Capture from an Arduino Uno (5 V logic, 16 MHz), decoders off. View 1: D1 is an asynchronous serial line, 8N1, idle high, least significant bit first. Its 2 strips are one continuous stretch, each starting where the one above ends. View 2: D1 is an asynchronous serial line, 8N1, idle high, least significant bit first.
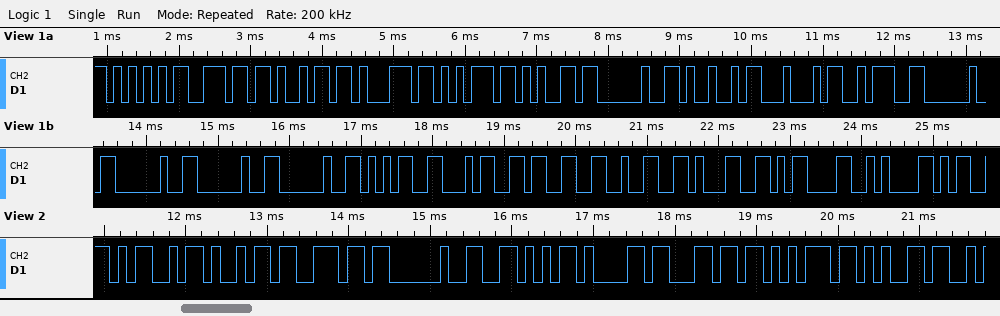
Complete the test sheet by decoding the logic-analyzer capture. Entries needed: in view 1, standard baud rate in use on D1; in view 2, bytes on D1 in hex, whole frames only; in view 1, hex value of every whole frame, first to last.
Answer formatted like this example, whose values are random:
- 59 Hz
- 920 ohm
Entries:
- 9600 baud
- 0x4D 0x69 0x6E 0x20 0x56 0x61 0x6C 0x75 0x65
- 55 6E 69 71 75 65 20 49 44 3A 20 20 20 20 35 34 33 32 31 0D 0A
